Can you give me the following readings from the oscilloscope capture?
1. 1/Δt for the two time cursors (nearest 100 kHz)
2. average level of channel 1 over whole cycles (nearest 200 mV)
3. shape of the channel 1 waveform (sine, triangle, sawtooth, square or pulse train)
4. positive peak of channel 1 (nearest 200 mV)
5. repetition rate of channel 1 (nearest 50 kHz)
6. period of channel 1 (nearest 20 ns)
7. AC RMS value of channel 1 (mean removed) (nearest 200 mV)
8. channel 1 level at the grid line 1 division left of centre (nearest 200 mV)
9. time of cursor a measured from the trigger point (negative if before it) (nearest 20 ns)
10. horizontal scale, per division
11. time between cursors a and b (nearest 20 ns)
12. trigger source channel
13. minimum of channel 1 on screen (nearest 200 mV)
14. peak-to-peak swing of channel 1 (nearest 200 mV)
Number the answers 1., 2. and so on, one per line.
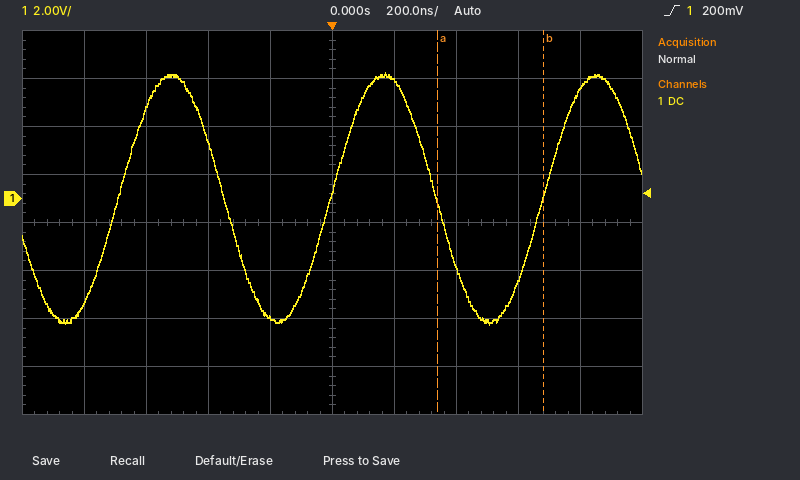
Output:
1. 2.9 MHz
2. 0.0 V
3. sine
4. 5.2 V
5. 1.45 MHz
6. 680 ns
7. 3.6 V
8. -5.0 V
9. +340 ns
10. 200 ns
11. 340 ns
12. channel 1
13. -5.2 V
14. 10.4 V
